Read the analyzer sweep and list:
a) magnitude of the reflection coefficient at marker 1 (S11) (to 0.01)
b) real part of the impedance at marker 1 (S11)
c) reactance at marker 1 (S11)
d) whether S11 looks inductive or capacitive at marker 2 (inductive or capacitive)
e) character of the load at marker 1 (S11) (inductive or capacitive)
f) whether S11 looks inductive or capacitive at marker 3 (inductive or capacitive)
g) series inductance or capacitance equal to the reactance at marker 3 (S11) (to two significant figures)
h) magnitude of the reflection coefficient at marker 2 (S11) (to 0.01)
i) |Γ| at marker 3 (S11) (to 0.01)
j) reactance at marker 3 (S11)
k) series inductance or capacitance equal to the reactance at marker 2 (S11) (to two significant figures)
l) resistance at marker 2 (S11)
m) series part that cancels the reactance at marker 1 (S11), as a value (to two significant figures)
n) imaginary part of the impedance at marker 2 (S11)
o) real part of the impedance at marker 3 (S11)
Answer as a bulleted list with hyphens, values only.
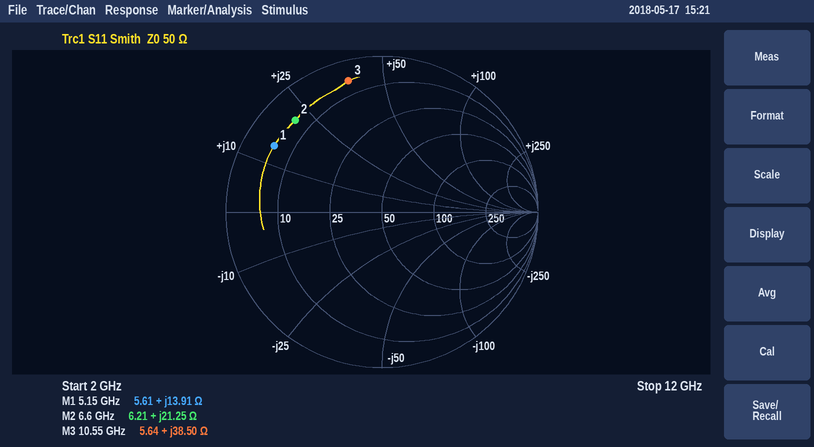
- 0.81
- 5.61 Ω
- +13.91 Ω
- inductive
- inductive
- inductive
- 580 pH
- 0.81
- 0.87
- +38.50 Ω
- 510 pH
- 6.21 Ω
- 2.2 pF
- +21.25 Ω
- 5.64 Ω
